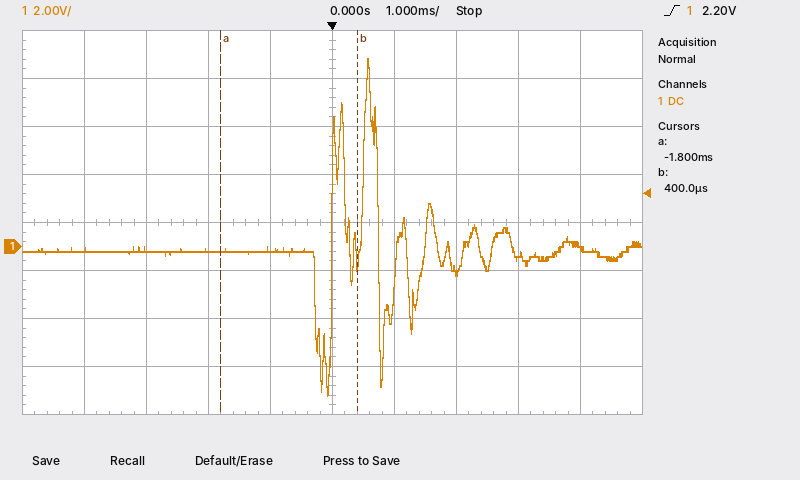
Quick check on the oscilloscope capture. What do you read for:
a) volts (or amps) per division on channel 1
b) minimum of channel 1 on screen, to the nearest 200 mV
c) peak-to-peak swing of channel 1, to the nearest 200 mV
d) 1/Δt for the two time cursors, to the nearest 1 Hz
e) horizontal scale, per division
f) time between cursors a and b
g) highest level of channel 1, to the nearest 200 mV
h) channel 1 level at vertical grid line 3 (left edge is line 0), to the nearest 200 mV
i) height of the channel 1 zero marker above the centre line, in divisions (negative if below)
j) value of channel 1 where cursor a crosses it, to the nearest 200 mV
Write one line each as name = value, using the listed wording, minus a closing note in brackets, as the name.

volts (or amps) per division on channel 1 = 2 V
minimum of channel 1 on screen, to the nearest 200 mV = -6.2 V
peak-to-peak swing of channel 1, to the nearest 200 mV = 14.0 V
1/Δt for the two time cursors, to the nearest 1 Hz = 455 Hz
horizontal scale, per division = 1 ms
time between cursors a and b = 2.2 ms
highest level of channel 1, to the nearest 200 mV = 7.8 V
channel 1 level at vertical grid line 3 (left edge is line 0), to the nearest 200 mV = -200 mV
height of the channel 1 zero marker above the centre line, in divisions = -0.5 div
value of channel 1 where cursor a crosses it, to the nearest 200 mV = -200 mV
